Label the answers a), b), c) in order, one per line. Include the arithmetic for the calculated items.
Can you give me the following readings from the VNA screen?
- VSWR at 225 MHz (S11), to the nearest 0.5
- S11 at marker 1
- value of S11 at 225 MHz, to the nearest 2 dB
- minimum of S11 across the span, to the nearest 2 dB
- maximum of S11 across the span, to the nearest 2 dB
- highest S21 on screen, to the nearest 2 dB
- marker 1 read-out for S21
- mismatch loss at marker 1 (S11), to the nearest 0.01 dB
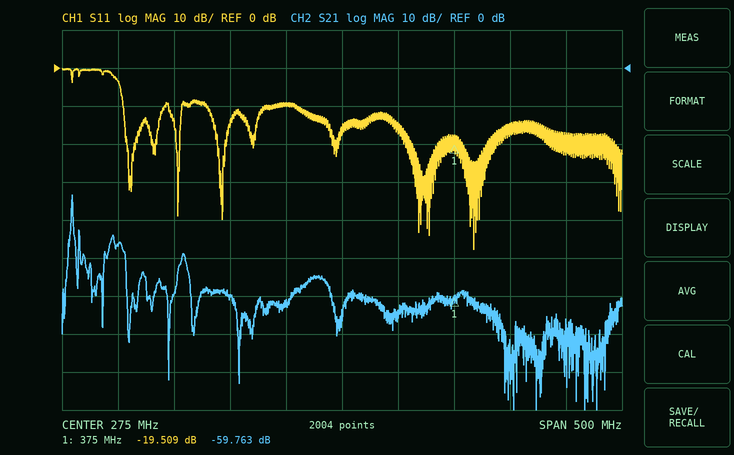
a) |Γ| = 10^(-10/20) = 0.3162; VSWR = (1 + 0.3162)/(1 − 0.3162) ≈ 1.92, so 2.0 to the nearest 0.5
b) -19.509 dB
c) -10 dB
d) -48 dB
e) 0 dB
f) -34 dB
g) -59.763 dB
h) −10 log10(1 − 10^(-19.509/10)) ≈ 0.05 dB
